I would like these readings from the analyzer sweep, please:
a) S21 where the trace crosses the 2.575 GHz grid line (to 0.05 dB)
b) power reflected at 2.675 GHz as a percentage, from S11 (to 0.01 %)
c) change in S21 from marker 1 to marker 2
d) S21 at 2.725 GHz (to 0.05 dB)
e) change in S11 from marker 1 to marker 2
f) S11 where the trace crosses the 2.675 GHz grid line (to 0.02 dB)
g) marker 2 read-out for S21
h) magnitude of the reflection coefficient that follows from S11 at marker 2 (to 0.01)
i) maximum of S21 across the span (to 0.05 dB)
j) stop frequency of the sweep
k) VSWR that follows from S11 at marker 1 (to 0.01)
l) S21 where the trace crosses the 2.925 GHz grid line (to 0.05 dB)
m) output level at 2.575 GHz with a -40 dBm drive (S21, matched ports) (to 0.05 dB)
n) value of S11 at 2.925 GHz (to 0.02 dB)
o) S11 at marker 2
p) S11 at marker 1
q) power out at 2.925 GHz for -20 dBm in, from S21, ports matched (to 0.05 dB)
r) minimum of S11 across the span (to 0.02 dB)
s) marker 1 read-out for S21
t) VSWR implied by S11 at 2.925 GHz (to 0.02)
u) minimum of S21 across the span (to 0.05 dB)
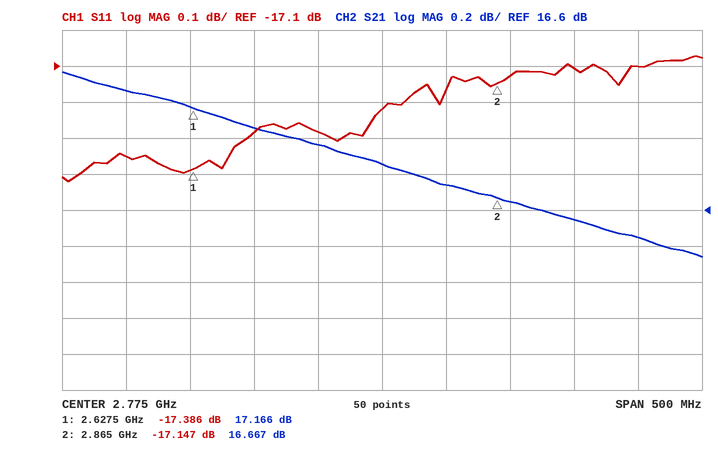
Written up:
17.25 dB
1.87 %
-0.499 dB
16.95 dB
0.239 dB
-17.28 dB
16.667 dB
0.14
17.35 dB
3.025 GHz
1.31
16.55 dB
-22.75 dBm
-17.10 dB
-17.147 dB
-17.386 dB
-3.45 dBm
-17.42 dB
17.166 dB
1.32
16.35 dB
